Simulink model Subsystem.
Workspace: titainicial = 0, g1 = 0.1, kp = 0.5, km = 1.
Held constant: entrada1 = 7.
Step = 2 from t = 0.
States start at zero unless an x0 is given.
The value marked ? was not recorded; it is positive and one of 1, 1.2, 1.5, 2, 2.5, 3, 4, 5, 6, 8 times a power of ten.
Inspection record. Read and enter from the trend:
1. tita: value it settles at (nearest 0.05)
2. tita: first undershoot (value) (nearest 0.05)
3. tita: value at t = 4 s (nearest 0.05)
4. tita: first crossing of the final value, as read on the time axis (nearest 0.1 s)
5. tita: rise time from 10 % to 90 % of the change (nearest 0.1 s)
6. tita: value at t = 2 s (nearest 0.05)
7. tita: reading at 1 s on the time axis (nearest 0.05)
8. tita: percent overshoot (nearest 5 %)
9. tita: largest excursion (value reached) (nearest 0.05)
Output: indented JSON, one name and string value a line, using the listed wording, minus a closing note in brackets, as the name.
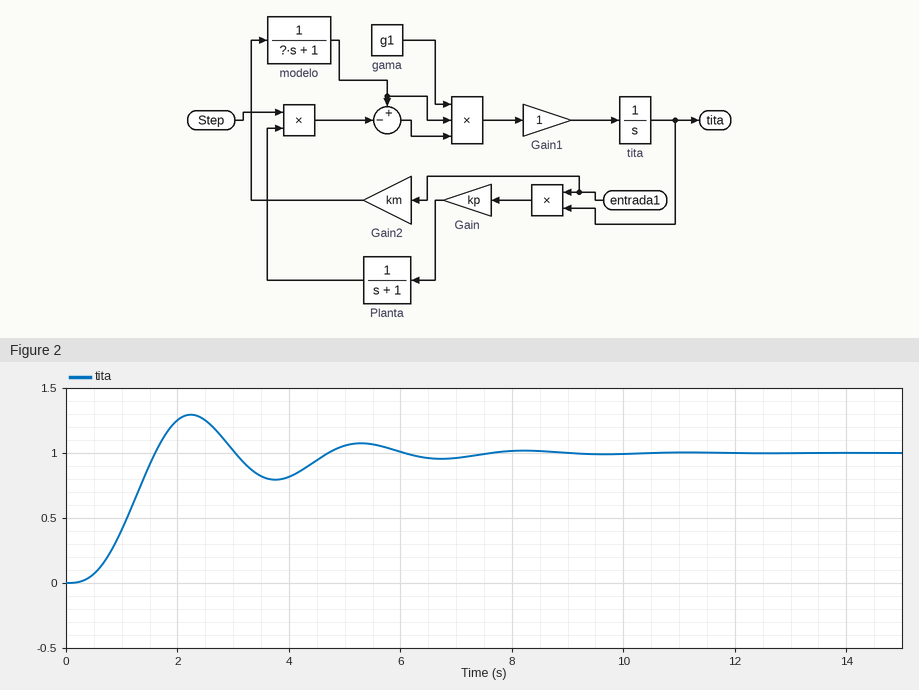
{
  "tita: value it settles at": "1.00",
  "tita: first undershoot (value)": "0.80",
  "tita: value at t = 4 s": "0.80",
  "tita: first crossing of the final value, as read on the time axis": "1.6 s",
  "tita: rise time from 10 % to 90 % of the change": "0.9 s",
  "tita: value at t = 2 s": "1.25",
  "tita: reading at 1 s on the time axis": "0.40",
  "tita: percent overshoot": "30 %",
  "tita: largest excursion (value reached)": "1.30"
}
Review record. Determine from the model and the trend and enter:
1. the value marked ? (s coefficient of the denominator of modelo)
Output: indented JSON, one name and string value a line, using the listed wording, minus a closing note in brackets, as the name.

{
  "the value marked ?": "1.5"
}
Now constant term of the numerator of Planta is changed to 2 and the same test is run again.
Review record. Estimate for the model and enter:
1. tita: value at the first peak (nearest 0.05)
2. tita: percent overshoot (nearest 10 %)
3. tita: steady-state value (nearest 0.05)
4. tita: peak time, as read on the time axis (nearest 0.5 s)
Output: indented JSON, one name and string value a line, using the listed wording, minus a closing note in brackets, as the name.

{
  "tita: value at the first peak": "0.70",
  "tita: percent overshoot": "40 %",
  "tita: steady-state value": "0.50",
  "tita: peak time, as read on the time axis": "1.5 s"
}
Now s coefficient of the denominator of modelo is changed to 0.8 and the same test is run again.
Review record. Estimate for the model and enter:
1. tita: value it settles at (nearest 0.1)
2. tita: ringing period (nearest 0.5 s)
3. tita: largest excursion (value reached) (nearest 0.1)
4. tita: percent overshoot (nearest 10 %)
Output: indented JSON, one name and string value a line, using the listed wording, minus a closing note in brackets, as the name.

{
  "tita: value it settles at": "1.0",
  "tita: ringing period": "3.0 s",
  "tita: largest excursion (value reached)": "1.7",
  "tita: percent overshoot": "70 %"
}
